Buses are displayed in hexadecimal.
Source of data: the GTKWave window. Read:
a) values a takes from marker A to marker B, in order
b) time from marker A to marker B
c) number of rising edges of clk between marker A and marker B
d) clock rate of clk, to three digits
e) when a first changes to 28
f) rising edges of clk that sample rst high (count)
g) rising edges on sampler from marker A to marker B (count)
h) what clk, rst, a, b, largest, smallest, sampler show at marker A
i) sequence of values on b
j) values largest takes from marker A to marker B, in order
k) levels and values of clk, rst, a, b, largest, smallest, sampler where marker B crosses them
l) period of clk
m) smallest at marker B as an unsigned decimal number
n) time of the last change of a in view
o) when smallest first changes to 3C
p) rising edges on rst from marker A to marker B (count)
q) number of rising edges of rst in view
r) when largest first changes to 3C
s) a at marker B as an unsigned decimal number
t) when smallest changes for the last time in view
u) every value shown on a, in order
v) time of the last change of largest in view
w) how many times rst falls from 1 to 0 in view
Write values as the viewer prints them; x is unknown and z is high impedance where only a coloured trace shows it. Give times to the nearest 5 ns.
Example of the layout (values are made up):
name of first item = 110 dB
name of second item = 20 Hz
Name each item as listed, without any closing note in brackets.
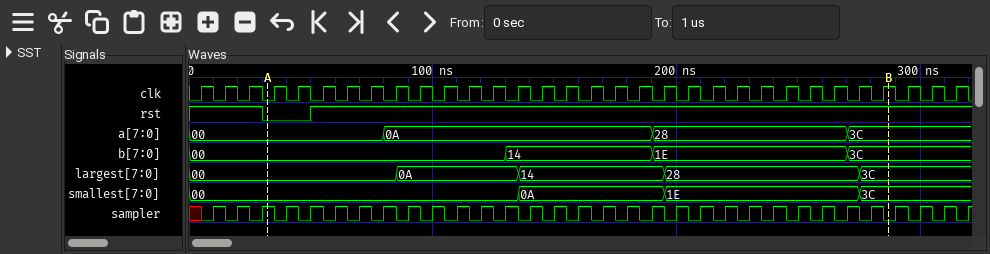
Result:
values a takes from marker A to marker B, in order = 00, 0A, 28, 3C
time from marker A to marker B = 255 ns
number of rising edges of clk between marker A and marker B = 26
clock rate of clk, to three digits = 100 MHz
when a first changes to 28 = 190 ns
rising edges of clk that sample rst high = 30
rising edges on sampler from marker A to marker B = 25
what clk, rst, a, b, largest, smallest, sampler show at marker A = clk=0, rst=0, a=00, b=00, largest=00, smallest=00, sampler=1
sequence of values on b = 00, 14, 1E, 3C
values largest takes from marker A to marker B, in order = 00, 0A, 14, 28, 3C
levels and values of clk, rst, a, b, largest, smallest, sampler where marker B crosses them = clk=1, rst=1, a=3C, b=3C, largest=3C, smallest=3C, sampler=0
period of clk = 10 ns
smallest at marker B as an unsigned decimal number = 60
time of the last change of a in view = 270 ns
when smallest first changes to 3C = 275 ns
rising edges on rst from marker A to marker B = 1
number of rising edges of rst in view = 1
when largest first changes to 3C = 275 ns
a at marker B as an unsigned decimal number = 60
when smallest changes for the last time in view = 275 ns
every value shown on a, in order = 00, 0A, 28, 3C
time of the last change of largest in view = 275 ns
how many times rst falls from 1 to 0 in view = 1
